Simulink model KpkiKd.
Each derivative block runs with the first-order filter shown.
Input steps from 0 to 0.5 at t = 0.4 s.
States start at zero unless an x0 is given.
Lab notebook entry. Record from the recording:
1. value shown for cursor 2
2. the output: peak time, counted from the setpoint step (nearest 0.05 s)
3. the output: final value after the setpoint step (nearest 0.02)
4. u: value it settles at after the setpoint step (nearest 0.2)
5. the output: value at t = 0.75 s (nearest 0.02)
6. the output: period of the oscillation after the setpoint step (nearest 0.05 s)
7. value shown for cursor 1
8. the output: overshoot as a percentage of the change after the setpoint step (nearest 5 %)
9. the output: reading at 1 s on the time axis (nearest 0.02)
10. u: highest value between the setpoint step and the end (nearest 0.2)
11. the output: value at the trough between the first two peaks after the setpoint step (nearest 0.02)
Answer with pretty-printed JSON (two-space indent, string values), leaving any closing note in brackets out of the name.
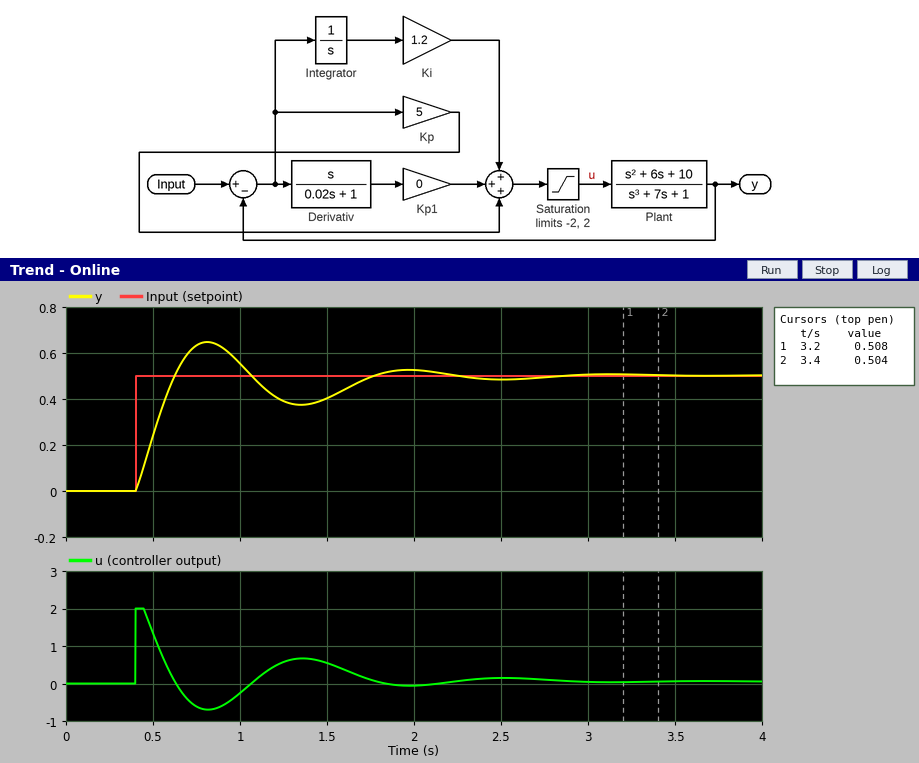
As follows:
{
  "value shown for cursor 2": "0.504",
  "the output: peak time, counted from the setpoint step": "0.40 s",
  "the output: final value after the setpoint step": "0.50",
  "u: value it settles at after the setpoint step": "0.0",
  "the output: value at t = 0.75 s": "0.64",
  "the output: period of the oscillation after the setpoint step": "1.15 s",
  "value shown for cursor 1": "0.508",
  "the output: overshoot as a percentage of the change after the setpoint step": "30 %",
  "the output: reading at 1 s on the time axis": "0.56",
  "u: highest value between the setpoint step and the end": "2.0",
  "the output: value at the trough between the first two peaks after the setpoint step": "0.38"
}
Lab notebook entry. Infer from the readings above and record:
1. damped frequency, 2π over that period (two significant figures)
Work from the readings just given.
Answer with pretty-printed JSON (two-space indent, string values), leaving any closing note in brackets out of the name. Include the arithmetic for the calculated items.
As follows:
{
  "damped frequency, 2π over that period": "2π / 1.15 = 5.5 rad/s"
}
